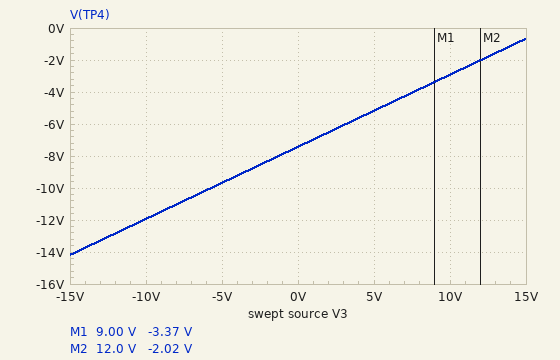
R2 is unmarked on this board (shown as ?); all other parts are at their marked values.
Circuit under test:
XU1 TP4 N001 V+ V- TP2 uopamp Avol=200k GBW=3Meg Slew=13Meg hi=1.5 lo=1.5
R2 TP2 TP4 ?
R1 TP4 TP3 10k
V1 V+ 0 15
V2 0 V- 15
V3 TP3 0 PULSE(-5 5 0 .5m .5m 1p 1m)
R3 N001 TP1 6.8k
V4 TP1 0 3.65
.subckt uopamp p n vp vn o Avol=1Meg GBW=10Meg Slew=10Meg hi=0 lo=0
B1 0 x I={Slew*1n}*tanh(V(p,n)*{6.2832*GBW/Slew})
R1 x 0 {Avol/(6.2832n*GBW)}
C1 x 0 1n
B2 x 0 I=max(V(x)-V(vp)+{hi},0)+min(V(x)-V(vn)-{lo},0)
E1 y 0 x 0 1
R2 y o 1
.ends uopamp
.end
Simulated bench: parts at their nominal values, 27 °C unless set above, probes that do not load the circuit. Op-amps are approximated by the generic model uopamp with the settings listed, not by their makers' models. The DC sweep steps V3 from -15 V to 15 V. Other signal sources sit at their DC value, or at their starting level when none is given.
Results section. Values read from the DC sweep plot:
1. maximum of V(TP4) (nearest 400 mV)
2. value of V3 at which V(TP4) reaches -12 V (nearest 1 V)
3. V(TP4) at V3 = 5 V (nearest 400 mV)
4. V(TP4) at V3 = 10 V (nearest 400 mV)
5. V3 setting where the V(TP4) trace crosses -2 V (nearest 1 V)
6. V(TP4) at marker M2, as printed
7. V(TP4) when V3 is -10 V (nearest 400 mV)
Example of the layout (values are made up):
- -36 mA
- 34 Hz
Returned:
- -800 mV
- -10 V
- -5.2 V
- -2.8 V
- 12 V
- -2.02 V
- -12.0 V
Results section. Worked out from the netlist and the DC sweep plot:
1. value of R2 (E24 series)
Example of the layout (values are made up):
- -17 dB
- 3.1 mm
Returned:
- 8.2 kΩ
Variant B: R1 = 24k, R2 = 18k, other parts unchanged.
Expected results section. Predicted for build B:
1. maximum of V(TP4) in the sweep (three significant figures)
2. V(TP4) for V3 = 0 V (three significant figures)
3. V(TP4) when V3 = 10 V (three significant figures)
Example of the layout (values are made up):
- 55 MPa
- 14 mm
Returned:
- -1.29 V
- -7.72 V
- -3.44 V
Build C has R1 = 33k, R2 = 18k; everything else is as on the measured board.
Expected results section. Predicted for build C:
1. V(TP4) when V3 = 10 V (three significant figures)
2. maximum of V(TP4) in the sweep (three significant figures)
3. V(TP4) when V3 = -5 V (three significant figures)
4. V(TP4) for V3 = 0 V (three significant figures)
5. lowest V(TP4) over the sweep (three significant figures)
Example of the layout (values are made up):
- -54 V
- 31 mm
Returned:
- -5.21 V
- -3.45 V
- -10.5 V
- -8.74 V
- -14.0 V
